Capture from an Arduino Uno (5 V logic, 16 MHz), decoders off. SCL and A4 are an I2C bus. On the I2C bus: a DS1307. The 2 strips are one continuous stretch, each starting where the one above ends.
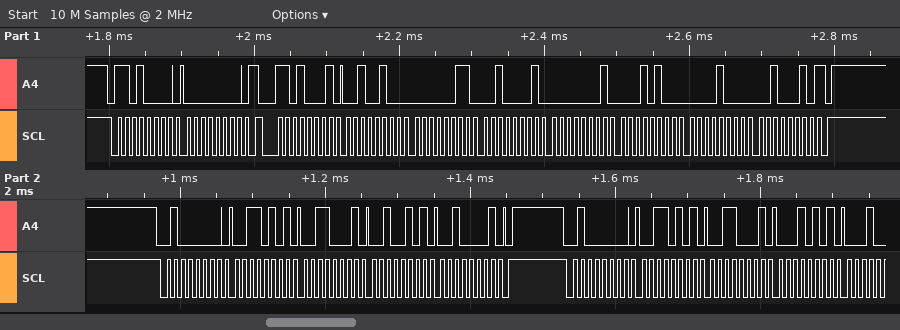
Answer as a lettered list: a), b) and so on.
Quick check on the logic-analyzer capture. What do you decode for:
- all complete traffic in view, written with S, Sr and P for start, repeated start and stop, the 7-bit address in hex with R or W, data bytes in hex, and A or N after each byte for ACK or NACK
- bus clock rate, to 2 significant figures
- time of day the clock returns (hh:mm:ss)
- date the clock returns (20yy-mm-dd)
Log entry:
a) S 68W A 00 A Sr 68R A 24 A 03 A 21 A 01 A 14 A 08 A 22 N P S 20W A 35 A 31 A 25 A 21 A P S 20W A 35 A 31 A 15 A
b) 100 kHz
c) 21:03:24
d) 2022-08-14
